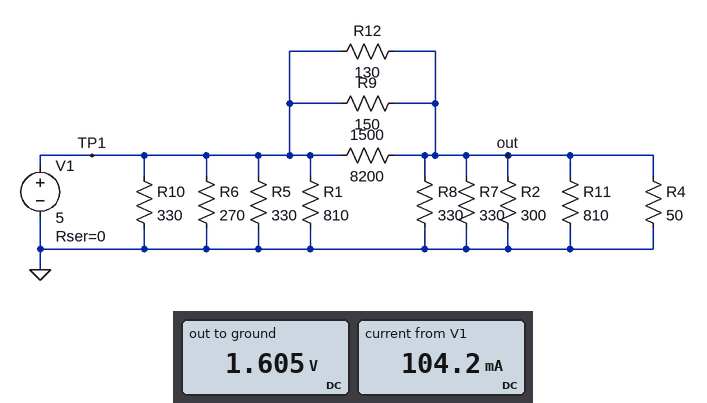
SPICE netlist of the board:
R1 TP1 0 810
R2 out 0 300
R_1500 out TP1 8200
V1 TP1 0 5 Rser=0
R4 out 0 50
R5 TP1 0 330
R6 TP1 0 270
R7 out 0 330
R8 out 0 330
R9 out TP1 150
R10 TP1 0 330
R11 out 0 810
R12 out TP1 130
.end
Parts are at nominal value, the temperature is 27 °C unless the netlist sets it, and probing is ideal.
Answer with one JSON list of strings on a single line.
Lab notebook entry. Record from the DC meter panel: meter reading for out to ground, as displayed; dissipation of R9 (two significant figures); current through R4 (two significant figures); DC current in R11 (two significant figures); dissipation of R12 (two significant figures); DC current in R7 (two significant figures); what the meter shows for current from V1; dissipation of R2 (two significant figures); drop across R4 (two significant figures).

["1.605 V", "77 mW", "32 mA", "2.0 mA", "89 mW", "4.9 mA", "104.2 mA", "8.6 mW", "1.6 V"]
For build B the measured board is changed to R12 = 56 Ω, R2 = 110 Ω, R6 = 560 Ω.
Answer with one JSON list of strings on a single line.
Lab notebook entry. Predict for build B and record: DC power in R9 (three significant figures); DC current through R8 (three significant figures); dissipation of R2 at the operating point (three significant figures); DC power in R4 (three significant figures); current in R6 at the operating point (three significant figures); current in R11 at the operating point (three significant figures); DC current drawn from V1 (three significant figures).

["59.2 mW", "6.12 mA", "37.1 mW", "81.5 mW", "8.93 mA", "2.49 mA", "119 mA"]
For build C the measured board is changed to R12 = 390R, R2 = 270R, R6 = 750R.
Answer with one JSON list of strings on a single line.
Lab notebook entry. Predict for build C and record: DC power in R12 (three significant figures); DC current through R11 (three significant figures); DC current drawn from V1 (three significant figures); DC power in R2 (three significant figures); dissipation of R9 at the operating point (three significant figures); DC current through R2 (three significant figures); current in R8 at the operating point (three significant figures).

["37.8 mW", "1.43 mA", "79.1 mA", "4.97 mW", "98.4 mW", "4.29 mA", "3.51 mA"]
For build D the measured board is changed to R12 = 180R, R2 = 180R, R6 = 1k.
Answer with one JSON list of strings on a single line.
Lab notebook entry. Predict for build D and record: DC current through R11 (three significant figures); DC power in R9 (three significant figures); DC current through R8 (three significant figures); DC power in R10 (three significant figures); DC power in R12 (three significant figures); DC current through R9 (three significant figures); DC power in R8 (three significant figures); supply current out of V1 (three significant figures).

["1.69 mA", "88.1 mW", "4.14 mA", "75.8 mW", "73.4 mW", "24.2 mA", "5.65 mW", "86.3 mA"]
